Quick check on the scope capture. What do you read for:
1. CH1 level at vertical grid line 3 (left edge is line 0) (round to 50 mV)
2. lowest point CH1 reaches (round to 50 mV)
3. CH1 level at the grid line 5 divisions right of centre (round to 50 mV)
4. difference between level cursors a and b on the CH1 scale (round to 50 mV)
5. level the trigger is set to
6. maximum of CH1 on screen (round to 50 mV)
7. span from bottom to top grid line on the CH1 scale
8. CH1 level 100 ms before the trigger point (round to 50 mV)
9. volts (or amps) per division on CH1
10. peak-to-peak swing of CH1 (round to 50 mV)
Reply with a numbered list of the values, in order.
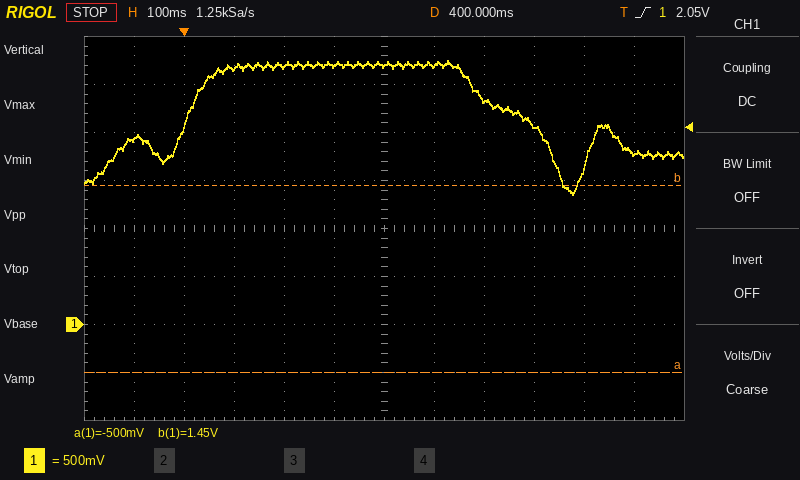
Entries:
1. 2.65 V
2. 1.35 V
3. 1.80 V
4. 1.95 V
5. 2.05 V
6. 2.75 V
7. 4 V
8. 1.95 V
9. 500 mV
10. 1.40 V
